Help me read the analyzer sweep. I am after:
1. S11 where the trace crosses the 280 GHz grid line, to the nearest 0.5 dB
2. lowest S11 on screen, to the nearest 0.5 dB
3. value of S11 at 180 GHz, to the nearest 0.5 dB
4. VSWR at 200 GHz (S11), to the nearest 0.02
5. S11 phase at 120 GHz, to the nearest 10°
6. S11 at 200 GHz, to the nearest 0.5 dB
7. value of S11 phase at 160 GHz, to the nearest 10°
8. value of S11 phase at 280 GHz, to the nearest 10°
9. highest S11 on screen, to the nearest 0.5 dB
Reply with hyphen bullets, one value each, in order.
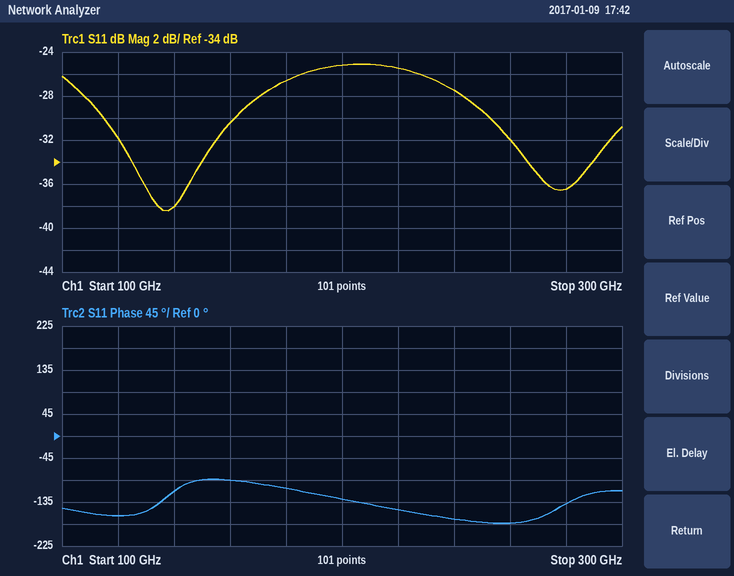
- -36.5 dB
- -38.5 dB
- -26.5 dB
- 1.12
- -160°
- -25.0 dB
- -90°
- -140°
- -25.0 dB
